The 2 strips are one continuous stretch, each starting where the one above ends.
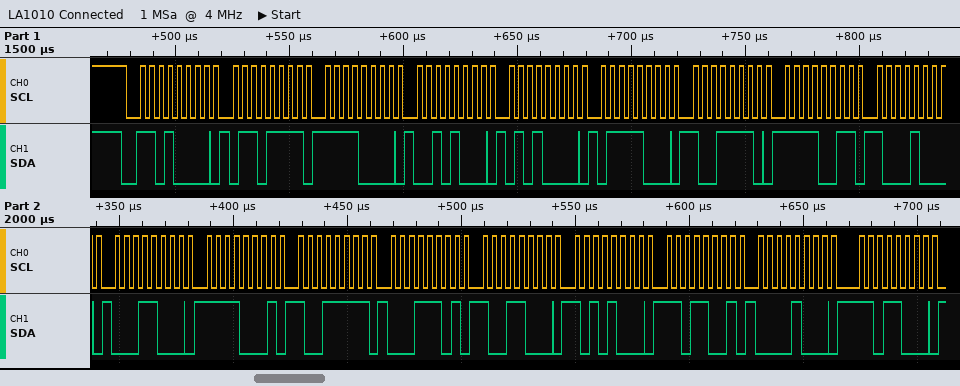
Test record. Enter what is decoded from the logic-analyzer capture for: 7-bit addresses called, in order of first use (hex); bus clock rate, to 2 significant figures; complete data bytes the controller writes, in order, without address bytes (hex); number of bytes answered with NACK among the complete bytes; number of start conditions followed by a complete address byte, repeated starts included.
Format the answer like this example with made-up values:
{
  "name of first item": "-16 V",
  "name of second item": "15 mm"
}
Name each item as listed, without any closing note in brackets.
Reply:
{
  "7-bit addresses called, in order of first use": "0x68",
  "bus clock rate, to 2 significant figures": "250 kHz",
  "complete data bytes the controller writes, in order, without address bytes": "6F F0 28 50 78 9E F3 88 18 F1 9F 1D 98 A8 D9 08 D8",
  "number of bytes answered with NACK among the complete bytes": "0",
  "number of start conditions followed by a complete address byte, repeated starts included": "1"
}
